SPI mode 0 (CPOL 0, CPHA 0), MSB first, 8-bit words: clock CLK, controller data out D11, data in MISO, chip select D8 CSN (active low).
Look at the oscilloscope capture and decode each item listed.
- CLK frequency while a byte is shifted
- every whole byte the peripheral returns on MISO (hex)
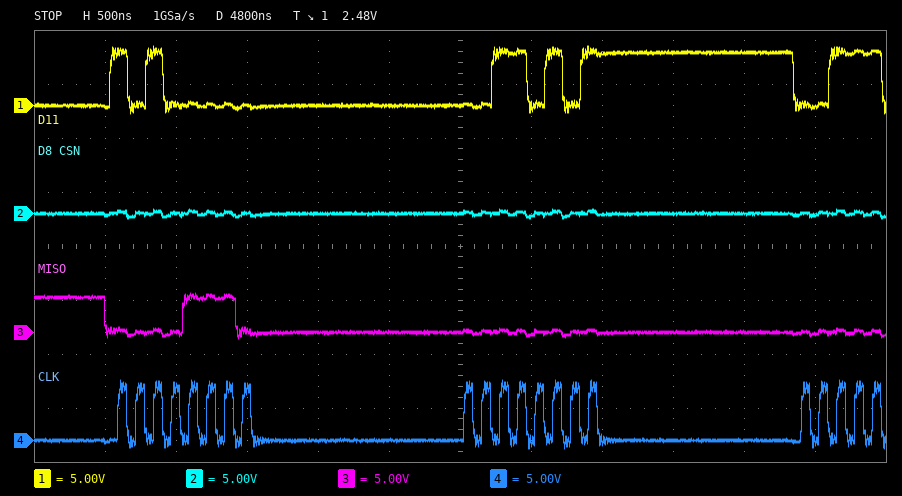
8 MHz
0E 00
